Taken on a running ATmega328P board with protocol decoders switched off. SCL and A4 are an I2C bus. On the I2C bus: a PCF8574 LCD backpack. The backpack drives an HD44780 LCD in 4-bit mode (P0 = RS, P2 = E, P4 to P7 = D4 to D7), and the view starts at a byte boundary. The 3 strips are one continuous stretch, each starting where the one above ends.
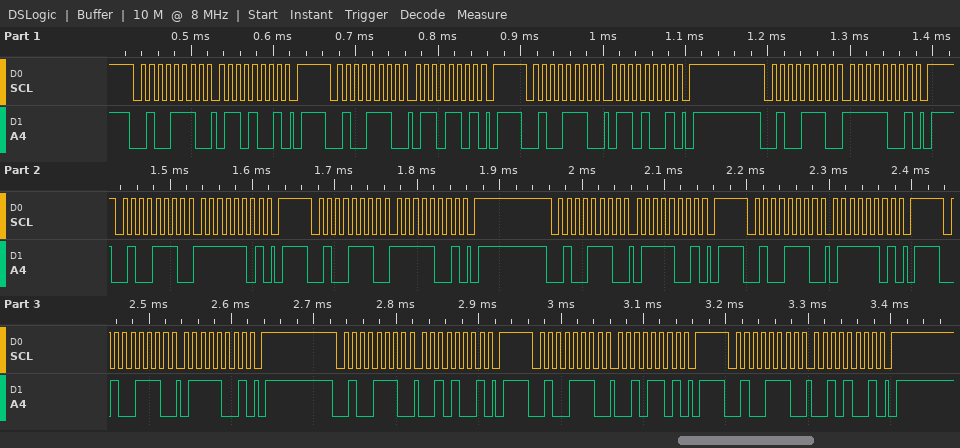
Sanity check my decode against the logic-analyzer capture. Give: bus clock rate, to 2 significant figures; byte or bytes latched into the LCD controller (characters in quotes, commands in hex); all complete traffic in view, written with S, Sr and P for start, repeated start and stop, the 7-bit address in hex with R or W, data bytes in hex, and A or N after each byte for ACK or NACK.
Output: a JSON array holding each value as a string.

["100 kHz", "'o' 'r'", "S 27W A 69 A P S 27W A 6D A P S 27W A 69 A P S 27W A F9 A P S 27W A FD A P S 27W A F9 A P S 27W A 79 A P S 27W A 7D A P S 27W A 79 A P S 27W A 29 A P S 27W A 2D A P S 27W A 29 A P"]
